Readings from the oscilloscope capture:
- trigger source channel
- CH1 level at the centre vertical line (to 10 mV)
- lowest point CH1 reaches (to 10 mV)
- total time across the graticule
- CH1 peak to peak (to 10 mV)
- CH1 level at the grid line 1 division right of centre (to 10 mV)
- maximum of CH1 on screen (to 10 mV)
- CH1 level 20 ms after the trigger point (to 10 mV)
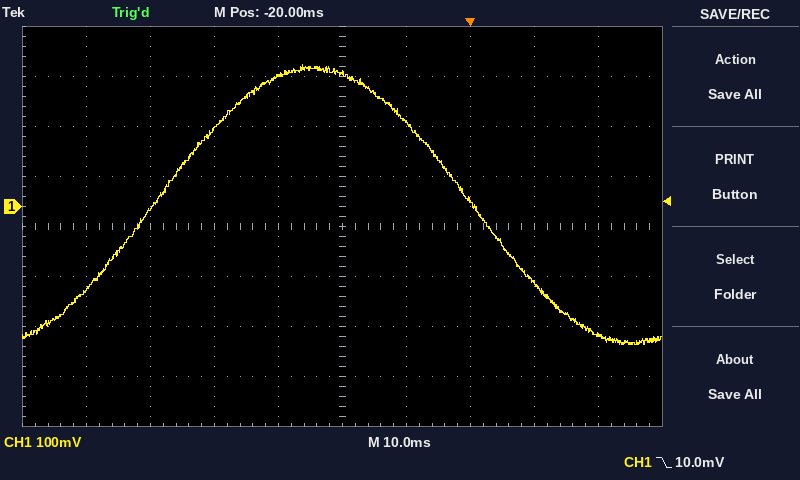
CH1
270 mV
-280 mV
100 ms
560 mV
170 mV
280 mV
-260 mV
